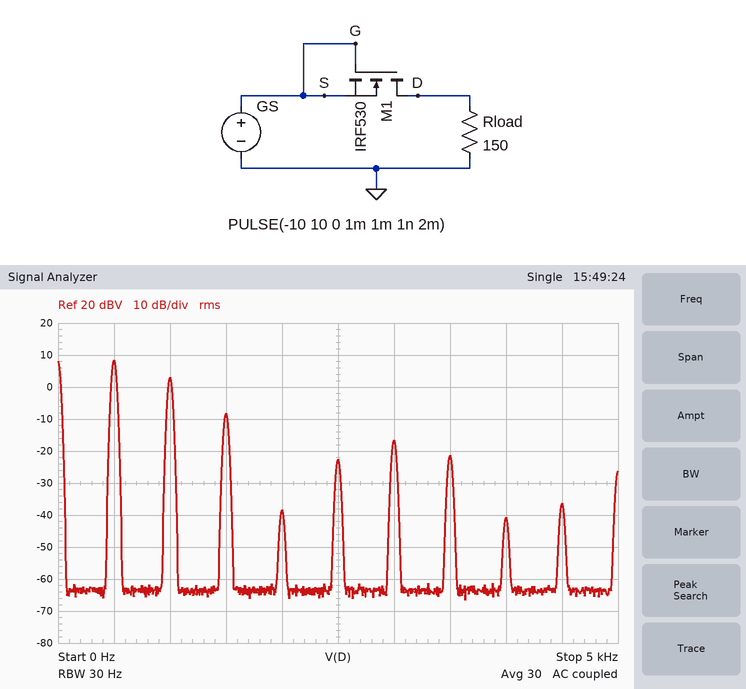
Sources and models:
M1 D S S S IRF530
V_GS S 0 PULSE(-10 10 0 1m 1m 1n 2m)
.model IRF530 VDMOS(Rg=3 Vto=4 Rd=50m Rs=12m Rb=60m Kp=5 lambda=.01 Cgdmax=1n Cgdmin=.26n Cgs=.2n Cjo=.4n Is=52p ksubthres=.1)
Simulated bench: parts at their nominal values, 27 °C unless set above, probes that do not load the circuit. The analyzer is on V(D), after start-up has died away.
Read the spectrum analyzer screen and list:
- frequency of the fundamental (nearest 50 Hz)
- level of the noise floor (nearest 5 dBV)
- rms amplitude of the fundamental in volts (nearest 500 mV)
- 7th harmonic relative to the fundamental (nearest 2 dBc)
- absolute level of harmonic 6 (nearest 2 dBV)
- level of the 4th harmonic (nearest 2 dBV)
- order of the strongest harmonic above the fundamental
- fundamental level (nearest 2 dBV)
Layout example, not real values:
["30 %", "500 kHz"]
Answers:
["500 Hz", "-65 dBV", "2.5 V", "-30 dBc", "-16 dBV", "-38 dBV", "2", "8 dBV"]
